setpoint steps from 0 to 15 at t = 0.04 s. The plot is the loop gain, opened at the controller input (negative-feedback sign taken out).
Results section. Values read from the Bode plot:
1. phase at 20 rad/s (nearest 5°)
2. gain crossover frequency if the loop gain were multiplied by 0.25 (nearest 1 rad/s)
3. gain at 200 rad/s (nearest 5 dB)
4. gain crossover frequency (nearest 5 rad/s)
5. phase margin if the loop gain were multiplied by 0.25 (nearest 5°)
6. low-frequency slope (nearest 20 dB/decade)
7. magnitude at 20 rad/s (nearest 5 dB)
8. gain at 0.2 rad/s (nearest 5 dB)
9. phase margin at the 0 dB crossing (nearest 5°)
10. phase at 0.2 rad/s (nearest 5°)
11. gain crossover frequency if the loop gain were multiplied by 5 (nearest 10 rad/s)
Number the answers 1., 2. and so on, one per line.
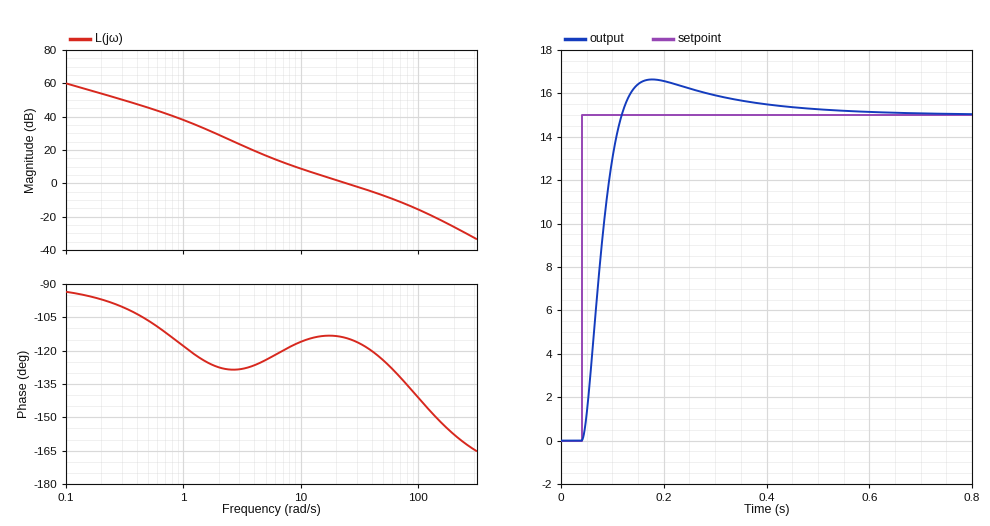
1. -115°
2. 7 rad/s
3. -25 dB
4. 25 rad/s
5. 60°
6. -20 dB/decade
7. 0 dB
8. 55 dB
9. 65°
10. -95°
11. 90 rad/s
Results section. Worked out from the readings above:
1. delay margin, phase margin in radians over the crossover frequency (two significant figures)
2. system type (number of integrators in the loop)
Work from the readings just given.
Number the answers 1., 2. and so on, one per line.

1. 0.045 s
2. 1
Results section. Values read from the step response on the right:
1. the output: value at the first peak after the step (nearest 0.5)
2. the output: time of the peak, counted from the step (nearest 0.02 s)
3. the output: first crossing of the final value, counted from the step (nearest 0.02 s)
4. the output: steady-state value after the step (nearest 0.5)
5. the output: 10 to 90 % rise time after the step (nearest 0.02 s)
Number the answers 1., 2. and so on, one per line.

1. 16.5
2. 0.14 s
3. 0.08 s
4. 15.0
5. 0.06 s
